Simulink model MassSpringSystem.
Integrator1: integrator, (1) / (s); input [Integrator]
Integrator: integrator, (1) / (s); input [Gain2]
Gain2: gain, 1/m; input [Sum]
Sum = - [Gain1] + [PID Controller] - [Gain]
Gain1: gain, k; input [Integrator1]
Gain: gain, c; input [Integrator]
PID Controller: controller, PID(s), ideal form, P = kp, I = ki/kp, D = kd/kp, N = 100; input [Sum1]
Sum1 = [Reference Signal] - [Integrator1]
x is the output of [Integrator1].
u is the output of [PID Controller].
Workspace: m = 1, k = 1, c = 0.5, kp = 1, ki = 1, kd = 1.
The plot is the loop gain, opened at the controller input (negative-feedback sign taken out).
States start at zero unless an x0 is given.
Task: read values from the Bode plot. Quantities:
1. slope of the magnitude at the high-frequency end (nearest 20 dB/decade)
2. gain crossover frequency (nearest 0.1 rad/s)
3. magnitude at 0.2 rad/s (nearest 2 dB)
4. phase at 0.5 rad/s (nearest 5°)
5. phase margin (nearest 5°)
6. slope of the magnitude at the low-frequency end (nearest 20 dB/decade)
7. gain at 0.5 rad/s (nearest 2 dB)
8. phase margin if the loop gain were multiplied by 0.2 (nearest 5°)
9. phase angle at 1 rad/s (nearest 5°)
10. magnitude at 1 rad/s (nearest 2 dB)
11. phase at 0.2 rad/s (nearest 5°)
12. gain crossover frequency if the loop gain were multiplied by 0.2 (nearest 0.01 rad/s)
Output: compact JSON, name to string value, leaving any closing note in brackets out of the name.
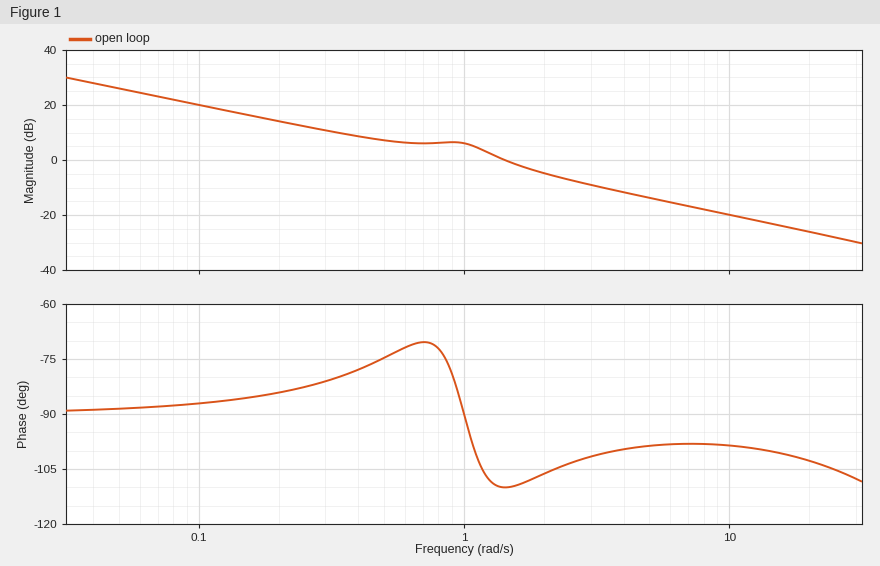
{"slope of the magnitude at the high-frequency end": "-20 dB/decade", "gain crossover frequency": "1.4 rad/s", "magnitude at 0.2 rad/s": "14 dB", "phase at 0.5 rad/s": "-75°", "phase margin": "70°", "slope of the magnitude at the low-frequency end": "-20 dB/decade", "gain at 0.5 rad/s": "8 dB", "phase margin if the loop gain were multiplied by 0.2": "95°", "phase angle at 1 rad/s": "-90°", "magnitude at 1 rad/s": "6 dB", "phase at 0.2 rad/s": "-85°", "gain crossover frequency if the loop gain were multiplied by 0.2": "0.20 rad/s"}
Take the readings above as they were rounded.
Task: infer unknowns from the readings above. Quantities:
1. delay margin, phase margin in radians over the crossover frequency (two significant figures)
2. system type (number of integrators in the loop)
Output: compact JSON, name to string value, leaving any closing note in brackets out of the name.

{"delay margin, phase margin in radians over the crossover frequency": "0.87 s", "system type": "1"}
